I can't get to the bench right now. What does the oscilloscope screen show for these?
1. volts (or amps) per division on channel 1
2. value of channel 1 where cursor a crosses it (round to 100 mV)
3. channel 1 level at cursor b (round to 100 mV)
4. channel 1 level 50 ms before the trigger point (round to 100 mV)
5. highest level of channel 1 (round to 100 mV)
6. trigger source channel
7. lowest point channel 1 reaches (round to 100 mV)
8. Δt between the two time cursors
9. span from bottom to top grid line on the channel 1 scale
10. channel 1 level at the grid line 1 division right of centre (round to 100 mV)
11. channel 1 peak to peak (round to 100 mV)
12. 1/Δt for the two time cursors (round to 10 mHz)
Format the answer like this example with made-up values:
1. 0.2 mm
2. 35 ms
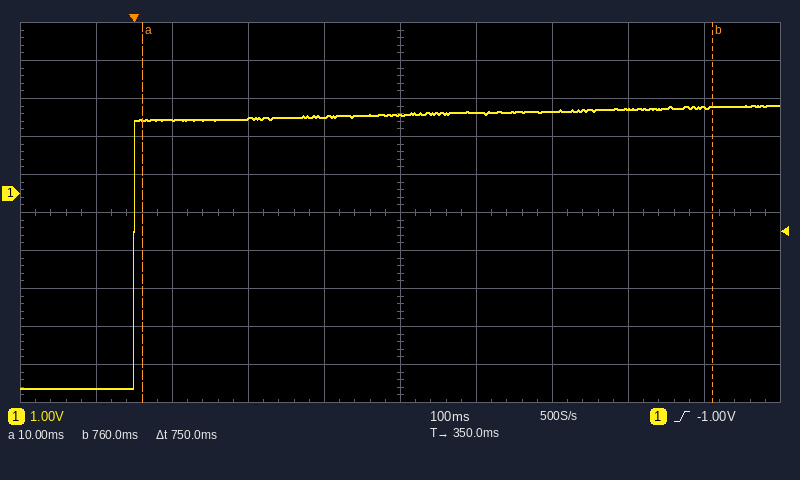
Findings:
1. 1 V
2. 1.9 V
3. 2.3 V
4. -5.1 V
5. 2.3 V
6. channel 1
7. -5.1 V
8. 750 ms
9. 10 V
10. 2.1 V
11. 7.4 V
12. 1.33 Hz
